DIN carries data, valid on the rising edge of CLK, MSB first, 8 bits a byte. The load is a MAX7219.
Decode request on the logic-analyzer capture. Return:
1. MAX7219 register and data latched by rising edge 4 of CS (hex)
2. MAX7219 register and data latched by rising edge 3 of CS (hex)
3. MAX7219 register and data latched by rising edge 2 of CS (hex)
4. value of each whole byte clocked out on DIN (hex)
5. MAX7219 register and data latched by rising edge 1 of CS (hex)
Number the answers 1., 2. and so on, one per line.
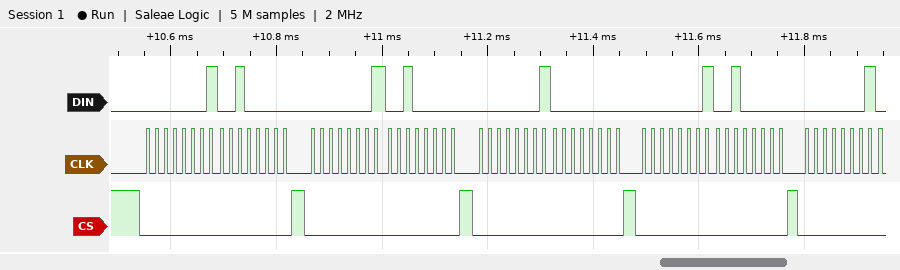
1. register 0x1, data 0x20
2. register 0x1, data 0x00
3. register 0x1, data 0x20
4. 01 20 01 20 01 00 01 20 01
5. register 0x1, data 0x20
